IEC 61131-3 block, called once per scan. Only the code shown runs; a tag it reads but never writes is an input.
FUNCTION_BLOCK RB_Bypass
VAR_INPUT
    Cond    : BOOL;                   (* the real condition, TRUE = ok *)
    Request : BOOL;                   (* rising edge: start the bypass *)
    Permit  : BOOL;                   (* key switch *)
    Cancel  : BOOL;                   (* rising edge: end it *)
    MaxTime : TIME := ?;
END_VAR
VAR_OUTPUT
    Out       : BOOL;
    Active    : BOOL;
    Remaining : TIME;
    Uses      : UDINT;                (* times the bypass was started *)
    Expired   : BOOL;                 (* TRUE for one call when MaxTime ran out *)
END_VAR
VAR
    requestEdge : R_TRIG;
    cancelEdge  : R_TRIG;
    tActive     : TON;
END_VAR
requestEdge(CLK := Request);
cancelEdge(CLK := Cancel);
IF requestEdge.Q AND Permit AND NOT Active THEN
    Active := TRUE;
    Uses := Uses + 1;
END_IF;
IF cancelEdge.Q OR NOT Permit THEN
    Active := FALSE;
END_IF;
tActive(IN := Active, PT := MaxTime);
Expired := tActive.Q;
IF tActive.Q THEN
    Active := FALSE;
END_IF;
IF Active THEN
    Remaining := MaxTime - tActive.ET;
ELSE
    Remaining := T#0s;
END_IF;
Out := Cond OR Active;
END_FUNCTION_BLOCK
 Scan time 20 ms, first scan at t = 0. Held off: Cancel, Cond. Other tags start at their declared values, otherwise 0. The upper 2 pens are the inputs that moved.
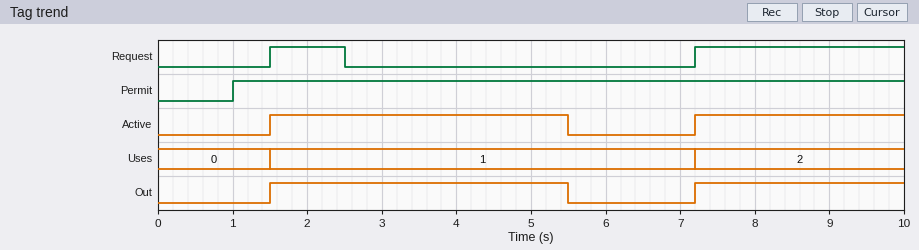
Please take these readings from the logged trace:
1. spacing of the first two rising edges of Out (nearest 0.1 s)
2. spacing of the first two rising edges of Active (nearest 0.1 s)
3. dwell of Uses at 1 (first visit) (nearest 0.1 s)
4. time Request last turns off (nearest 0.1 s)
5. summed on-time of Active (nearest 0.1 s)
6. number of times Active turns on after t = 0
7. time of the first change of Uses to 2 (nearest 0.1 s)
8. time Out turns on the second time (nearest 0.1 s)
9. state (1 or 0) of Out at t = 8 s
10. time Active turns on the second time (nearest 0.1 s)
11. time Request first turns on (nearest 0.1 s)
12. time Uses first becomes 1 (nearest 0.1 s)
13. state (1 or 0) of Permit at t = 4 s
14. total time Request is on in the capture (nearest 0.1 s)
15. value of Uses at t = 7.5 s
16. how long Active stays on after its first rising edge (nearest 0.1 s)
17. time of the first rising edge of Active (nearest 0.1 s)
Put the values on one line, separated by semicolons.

5.7 s; 5.7 s; 5.7 s; 2.5 s; 6.8 s; 2; 7.2 s; 7.2 s; 1; 7.2 s; 1.5 s; 1.5 s; 1; 3.8 s; 2; 4.0 s; 1.5 s
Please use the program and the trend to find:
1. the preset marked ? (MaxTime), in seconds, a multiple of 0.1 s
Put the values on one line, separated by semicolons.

4.0 s
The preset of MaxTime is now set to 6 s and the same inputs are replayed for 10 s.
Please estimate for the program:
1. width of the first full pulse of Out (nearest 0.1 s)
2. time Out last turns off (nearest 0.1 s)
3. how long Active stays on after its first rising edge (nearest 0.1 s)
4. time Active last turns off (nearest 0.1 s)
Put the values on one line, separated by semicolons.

6.0 s; 7.5 s; 6.0 s; 7.5 s
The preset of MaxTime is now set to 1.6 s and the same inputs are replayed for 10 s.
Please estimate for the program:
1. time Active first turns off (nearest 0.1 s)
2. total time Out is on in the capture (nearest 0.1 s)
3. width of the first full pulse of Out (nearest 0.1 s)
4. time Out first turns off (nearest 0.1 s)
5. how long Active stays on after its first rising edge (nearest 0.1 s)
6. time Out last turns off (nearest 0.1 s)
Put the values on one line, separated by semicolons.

3.1 s; 3.2 s; 1.6 s; 3.1 s; 1.6 s; 8.8 s
